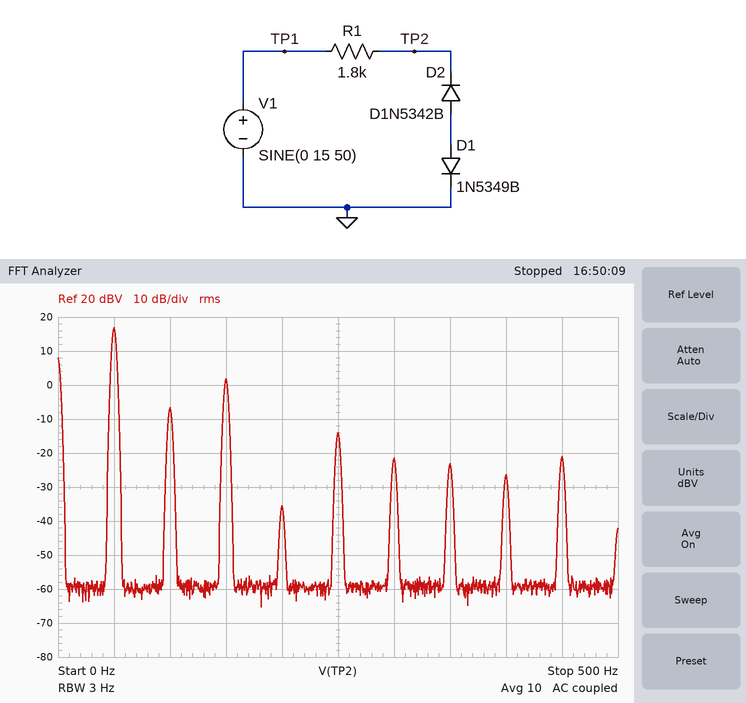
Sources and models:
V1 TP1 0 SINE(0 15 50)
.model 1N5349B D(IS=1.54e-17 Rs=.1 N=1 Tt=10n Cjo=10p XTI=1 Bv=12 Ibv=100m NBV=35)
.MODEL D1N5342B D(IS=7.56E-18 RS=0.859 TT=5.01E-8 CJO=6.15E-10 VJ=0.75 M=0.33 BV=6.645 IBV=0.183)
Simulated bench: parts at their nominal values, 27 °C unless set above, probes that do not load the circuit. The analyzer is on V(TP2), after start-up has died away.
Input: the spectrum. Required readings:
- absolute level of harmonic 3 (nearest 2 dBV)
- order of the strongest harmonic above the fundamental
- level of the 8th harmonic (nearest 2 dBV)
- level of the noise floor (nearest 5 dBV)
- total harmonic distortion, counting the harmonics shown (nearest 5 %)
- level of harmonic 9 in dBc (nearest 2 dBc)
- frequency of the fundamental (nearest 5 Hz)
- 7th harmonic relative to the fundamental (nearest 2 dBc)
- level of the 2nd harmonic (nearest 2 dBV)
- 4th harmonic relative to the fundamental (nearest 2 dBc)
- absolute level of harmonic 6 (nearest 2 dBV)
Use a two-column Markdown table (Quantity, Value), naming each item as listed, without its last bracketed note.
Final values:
| Quantity | Value |
|---|---|
| absolute level of harmonic 3 | 2 dBV |
| order of the strongest harmonic above the fundamental | 3 |
| level of the 8th harmonic | -26 dBV |
| level of the noise floor | -60 dBV |
| total harmonic distortion, counting the harmonics shown | 20 % |
| level of harmonic 9 in dBc | -38 dBc |
| frequency of the fundamental | 50 Hz |
| 7th harmonic relative to the fundamental | -40 dBc |
| level of the 2nd harmonic | -6 dBV |
| 4th harmonic relative to the fundamental | -52 dBc |
| absolute level of harmonic 6 | -22 dBV |
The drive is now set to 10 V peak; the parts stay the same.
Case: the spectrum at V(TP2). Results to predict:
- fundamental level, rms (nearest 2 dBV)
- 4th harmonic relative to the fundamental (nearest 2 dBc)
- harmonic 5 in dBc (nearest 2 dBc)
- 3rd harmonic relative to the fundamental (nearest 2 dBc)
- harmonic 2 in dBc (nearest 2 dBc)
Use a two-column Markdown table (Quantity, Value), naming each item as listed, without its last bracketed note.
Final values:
| Quantity | Value |
|---|---|
| fundamental level, rms | 16 dBV |
| 4th harmonic relative to the fundamental | -34 dBc |
| harmonic 5 in dBc | -34 dBc |
| 3rd harmonic relative to the fundamental | -22 dBc |
| harmonic 2 in dBc | -30 dBc |
